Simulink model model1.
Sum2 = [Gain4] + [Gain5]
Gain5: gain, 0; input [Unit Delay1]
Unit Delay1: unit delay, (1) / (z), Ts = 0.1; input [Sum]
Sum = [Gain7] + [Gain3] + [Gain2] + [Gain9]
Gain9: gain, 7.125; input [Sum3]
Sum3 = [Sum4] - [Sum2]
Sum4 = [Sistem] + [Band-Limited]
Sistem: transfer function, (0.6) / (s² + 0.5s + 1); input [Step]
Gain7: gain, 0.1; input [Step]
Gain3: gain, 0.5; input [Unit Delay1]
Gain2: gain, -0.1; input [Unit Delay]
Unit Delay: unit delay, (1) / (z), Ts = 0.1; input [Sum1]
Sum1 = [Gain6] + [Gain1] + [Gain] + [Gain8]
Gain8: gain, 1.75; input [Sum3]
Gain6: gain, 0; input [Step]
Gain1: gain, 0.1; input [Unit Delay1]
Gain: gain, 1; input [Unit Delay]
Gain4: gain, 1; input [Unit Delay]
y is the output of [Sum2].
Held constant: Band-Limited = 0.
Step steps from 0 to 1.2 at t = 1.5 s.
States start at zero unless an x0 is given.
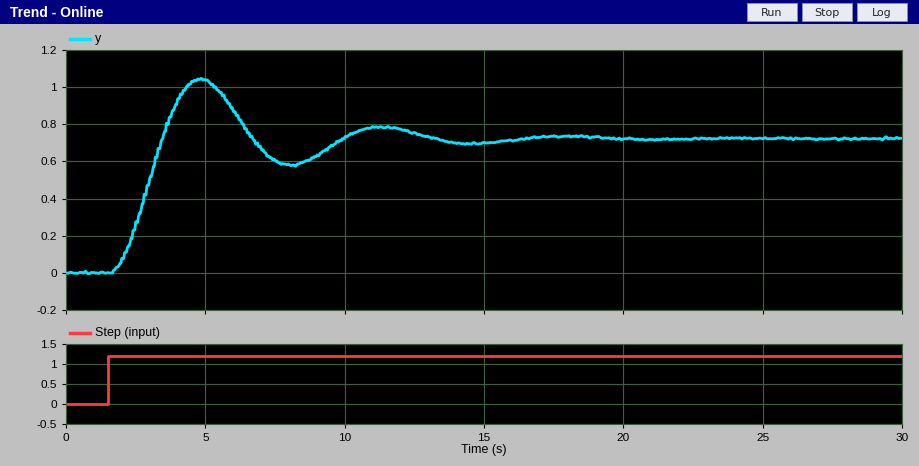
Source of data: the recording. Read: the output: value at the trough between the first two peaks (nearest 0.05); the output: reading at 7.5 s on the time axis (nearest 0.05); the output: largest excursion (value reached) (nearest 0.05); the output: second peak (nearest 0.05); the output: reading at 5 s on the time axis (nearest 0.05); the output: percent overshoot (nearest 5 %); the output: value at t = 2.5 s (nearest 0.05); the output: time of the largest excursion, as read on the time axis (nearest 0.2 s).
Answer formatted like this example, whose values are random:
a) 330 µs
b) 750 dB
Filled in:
a) 0.60
b) 0.60
c) 1.05
d) 0.80
e) 1.05
f) 45 %
g) 0.25
h) 4.8 s
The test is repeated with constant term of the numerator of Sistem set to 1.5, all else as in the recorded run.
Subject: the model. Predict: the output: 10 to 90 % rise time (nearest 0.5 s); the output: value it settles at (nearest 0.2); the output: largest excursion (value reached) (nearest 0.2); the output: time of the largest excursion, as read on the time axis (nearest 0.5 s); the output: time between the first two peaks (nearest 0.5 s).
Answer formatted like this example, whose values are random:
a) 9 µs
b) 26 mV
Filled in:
a) 1.5 s
b) 1.8
c) 2.6
d) 5.0 s
e) 6.5 s
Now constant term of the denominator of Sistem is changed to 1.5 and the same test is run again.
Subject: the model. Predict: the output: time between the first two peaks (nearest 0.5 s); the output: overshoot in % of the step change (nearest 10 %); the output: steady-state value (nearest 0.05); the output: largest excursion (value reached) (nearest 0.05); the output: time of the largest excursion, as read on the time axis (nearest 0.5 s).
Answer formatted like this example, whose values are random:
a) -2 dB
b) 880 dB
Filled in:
a) 5.5 s
b) 50 %
c) 0.50
d) 0.75
e) 4.0 s
